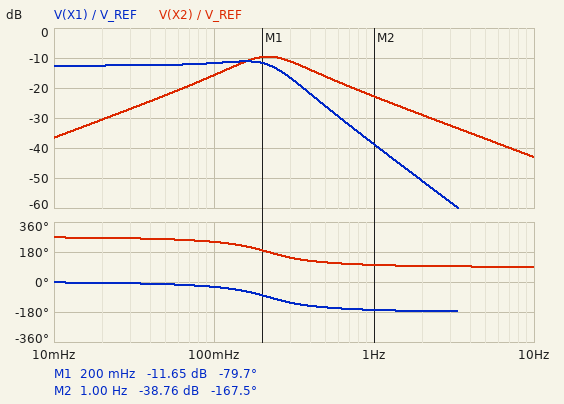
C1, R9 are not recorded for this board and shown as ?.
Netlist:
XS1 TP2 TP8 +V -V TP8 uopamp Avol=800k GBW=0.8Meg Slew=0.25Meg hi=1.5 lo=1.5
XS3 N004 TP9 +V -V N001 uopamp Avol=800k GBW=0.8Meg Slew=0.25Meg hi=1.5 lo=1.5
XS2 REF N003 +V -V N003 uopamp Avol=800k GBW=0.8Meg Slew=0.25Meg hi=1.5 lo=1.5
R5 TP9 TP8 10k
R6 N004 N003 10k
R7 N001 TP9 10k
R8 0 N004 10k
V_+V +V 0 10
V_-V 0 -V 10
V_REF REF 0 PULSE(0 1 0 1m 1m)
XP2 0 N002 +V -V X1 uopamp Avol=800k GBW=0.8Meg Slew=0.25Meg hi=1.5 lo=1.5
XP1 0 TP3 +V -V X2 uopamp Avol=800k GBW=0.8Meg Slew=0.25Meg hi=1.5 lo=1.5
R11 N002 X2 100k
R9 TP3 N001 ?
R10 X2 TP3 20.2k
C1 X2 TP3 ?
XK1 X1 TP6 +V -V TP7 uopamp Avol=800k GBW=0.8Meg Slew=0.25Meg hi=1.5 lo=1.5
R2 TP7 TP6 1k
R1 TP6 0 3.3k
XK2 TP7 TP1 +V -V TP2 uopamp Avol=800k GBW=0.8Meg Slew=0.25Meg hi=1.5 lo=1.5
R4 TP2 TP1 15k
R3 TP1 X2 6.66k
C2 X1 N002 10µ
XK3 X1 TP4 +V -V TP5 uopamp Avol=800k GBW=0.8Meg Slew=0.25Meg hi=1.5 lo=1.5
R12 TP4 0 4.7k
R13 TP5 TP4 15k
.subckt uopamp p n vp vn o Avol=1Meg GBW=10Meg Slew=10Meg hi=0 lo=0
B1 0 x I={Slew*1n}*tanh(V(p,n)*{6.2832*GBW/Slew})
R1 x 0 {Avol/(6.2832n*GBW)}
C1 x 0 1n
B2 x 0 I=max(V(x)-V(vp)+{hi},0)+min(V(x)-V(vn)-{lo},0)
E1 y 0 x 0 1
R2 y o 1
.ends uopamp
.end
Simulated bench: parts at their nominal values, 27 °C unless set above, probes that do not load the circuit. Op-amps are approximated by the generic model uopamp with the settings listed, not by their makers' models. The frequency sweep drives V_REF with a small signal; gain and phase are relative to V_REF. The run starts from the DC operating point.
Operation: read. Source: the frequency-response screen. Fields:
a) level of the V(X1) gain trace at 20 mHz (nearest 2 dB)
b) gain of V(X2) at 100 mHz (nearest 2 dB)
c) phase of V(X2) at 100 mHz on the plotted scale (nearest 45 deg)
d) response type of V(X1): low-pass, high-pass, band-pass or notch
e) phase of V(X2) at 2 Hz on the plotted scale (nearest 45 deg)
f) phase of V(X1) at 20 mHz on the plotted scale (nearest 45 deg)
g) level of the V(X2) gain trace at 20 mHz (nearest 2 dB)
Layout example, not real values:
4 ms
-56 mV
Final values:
-12 dB
-16 dB
225 deg
low-pass
90 deg
0 deg
-30 dB
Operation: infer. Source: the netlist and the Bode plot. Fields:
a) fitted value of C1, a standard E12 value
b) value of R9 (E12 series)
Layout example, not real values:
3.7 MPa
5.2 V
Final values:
150 µF
15 kΩ
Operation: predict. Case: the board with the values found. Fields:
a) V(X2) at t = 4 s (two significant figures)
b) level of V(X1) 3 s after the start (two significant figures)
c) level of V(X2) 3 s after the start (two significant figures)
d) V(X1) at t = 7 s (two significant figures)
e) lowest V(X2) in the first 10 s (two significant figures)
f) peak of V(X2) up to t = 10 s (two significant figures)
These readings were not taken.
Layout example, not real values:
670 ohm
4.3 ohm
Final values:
26 mV
270 mV
22 mV
240 mV
-180 mV
31 mV
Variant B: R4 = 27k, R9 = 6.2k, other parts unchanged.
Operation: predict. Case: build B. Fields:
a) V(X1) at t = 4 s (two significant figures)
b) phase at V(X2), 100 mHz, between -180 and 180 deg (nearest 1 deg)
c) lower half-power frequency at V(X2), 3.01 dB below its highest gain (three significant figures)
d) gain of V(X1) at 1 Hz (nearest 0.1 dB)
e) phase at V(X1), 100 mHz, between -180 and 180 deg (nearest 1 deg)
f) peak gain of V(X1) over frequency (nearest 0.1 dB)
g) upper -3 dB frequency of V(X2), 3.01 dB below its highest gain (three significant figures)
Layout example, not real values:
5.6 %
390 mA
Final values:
150 mV
-114 deg
191 mHz
-32.2 dB
-24 deg
-16.4 dB
938 mHz
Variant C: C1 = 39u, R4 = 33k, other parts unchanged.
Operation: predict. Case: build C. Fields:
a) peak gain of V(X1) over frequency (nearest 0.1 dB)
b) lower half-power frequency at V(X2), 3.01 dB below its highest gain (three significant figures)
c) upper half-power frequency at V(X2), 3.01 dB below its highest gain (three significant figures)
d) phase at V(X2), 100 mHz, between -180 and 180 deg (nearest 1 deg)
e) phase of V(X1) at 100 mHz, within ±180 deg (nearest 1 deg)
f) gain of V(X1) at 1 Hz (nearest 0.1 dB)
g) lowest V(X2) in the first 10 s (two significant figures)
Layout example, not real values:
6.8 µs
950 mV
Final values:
-17.8 dB
193 mHz
1.74 Hz
-115 deg
-25 deg
-31.8 dB
-140 mV
